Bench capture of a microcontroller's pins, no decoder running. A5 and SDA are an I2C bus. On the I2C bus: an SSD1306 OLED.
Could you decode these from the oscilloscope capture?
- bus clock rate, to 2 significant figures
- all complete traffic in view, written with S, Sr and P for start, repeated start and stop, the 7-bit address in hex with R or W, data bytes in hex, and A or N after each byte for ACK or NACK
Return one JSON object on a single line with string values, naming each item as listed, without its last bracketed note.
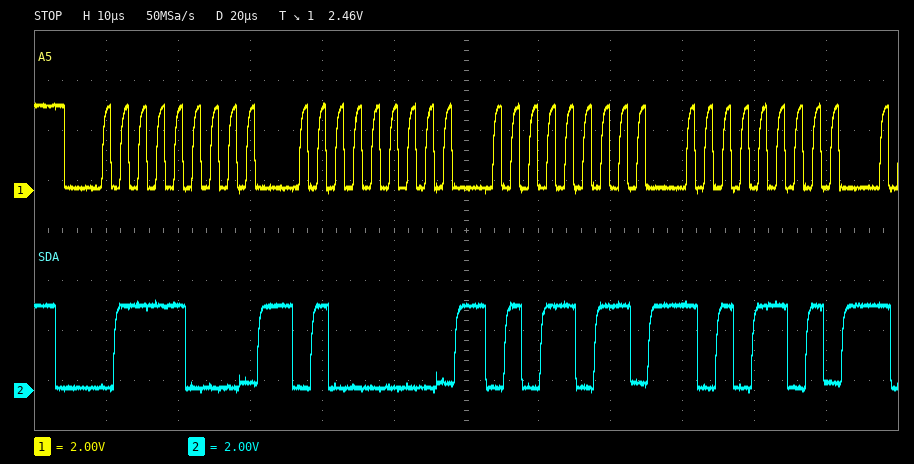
{"bus clock rate, to 2 significant figures": "400 kHz", "all complete traffic in view, written with S, Sr and P for start, repeated start and stop, the 7-bit address in hex with R or W, data bytes in hex, and A or N after each byte for ACK or NACK": "S 3CW A 40 A 5B A AD A"}
